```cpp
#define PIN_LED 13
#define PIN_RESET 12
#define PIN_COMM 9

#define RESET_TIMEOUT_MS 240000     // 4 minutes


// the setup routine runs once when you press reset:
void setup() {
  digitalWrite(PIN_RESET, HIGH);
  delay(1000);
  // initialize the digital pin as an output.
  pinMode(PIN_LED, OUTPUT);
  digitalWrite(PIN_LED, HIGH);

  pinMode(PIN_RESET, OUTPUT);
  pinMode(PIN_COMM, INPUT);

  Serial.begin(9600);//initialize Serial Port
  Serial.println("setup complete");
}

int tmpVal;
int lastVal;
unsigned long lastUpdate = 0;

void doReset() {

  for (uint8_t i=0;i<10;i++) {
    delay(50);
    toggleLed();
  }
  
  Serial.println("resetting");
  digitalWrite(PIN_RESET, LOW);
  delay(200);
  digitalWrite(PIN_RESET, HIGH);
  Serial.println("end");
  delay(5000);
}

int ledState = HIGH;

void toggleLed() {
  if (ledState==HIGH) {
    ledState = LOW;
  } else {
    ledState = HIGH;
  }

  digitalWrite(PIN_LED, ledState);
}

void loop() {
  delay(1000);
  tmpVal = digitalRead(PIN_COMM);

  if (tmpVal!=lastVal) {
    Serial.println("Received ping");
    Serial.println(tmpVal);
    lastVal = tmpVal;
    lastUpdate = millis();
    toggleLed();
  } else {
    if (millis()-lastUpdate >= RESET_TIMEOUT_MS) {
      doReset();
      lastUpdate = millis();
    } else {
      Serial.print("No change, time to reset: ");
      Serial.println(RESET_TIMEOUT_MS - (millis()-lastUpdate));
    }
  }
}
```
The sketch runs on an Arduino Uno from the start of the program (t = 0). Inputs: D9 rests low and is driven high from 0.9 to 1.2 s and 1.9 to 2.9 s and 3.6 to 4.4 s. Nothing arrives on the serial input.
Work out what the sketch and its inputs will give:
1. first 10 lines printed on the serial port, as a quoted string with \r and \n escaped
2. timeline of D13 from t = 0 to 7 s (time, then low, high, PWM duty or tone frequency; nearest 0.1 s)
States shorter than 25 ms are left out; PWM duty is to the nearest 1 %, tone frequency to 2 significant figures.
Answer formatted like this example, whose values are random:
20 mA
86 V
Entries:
"setup complete\r\nReceived ping\r\n1\r\nReceived ping\r\n0\r\nReceived ping\r\n1\r\nReceived ping\r\n0\r\nNo change, time to reset: 239000\r\n"
1 s high; 2 s low; 3 s high; 4 s low; 5 s high
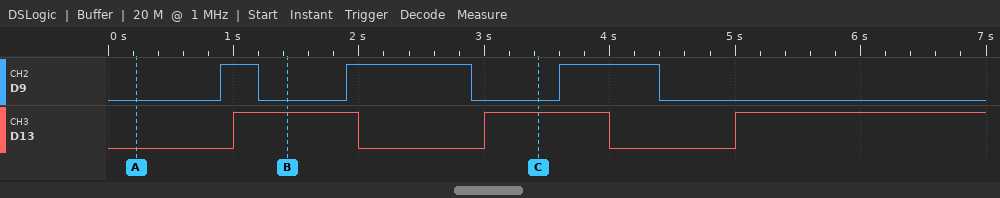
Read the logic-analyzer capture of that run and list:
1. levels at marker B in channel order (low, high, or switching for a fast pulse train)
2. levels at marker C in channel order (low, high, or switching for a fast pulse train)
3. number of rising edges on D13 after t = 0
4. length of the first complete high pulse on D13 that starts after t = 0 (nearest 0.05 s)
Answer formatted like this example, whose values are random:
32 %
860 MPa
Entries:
D9 low, D13 high
D9 low, D13 high
3
1.00 s
